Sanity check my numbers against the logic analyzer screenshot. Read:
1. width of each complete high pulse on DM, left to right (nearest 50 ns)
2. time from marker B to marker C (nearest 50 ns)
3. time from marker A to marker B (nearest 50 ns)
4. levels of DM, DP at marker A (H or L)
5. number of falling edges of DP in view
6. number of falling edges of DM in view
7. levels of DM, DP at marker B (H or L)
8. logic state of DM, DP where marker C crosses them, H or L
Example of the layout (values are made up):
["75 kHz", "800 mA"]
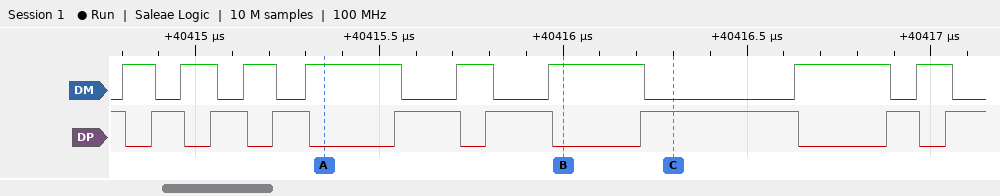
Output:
["100 ns, 100 ns, 100 ns, 250 ns, 100 ns, 250 ns, 250 ns, 100 ns", "300 ns", "650 ns", "DM=H, DP=L", "8", "8", "DM=H, DP=L", "DM=L, DP=H"]
